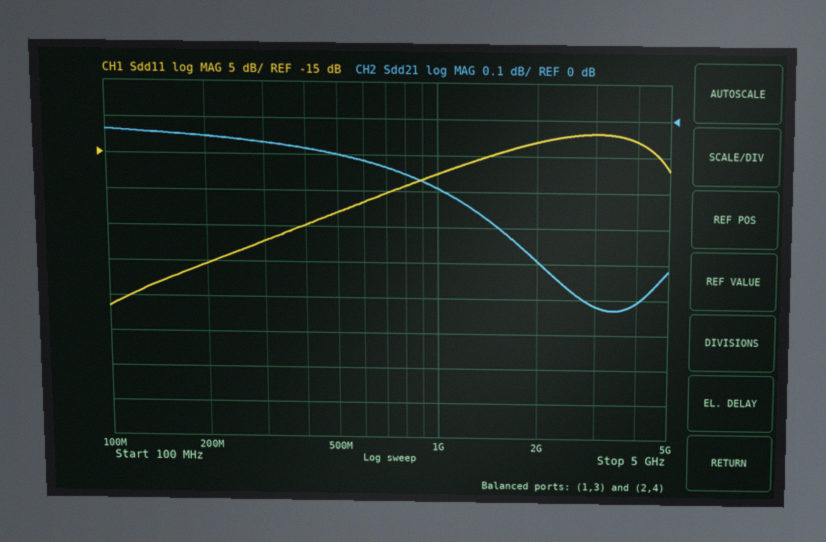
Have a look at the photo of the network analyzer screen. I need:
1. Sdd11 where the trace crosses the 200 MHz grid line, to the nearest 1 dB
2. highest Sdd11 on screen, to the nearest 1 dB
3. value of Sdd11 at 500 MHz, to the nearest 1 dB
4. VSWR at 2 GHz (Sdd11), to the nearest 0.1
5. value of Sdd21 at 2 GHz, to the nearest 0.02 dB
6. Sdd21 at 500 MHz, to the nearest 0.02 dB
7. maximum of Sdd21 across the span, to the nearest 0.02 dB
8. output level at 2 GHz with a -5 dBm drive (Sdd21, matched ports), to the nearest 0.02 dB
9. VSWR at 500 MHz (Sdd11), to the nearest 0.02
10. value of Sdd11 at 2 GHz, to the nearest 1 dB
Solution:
-30 dB
-12 dB
-23 dB
1.6
-0.40 dB
-0.10 dB
-0.04 dB
-5.40 dBm
1.16
-13 dB
